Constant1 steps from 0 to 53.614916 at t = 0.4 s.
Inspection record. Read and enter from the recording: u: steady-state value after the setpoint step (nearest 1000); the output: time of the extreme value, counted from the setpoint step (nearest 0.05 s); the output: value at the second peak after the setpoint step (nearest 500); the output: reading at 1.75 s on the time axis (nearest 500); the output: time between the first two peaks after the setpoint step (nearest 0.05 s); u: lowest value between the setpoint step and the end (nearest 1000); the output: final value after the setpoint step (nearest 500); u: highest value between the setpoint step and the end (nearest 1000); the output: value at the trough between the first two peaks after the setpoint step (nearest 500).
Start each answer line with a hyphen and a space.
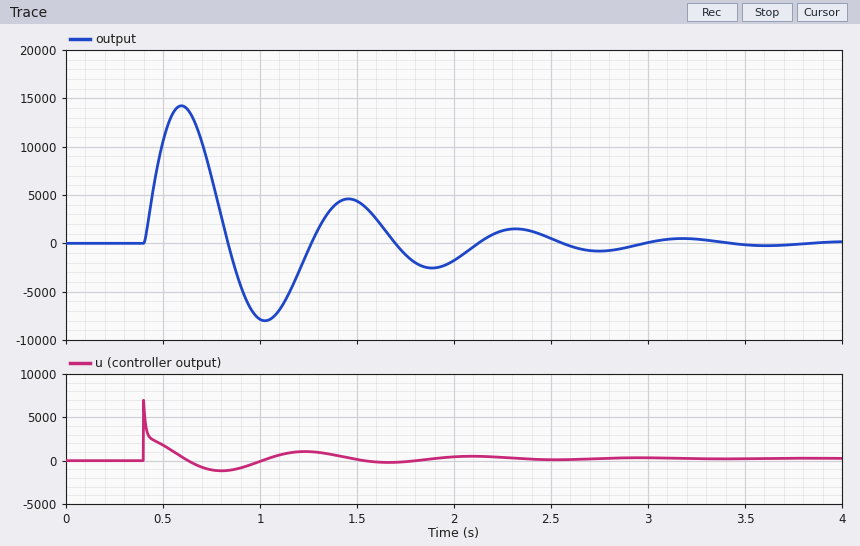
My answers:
- 0
- 0.20 s
- 4500
- -1000
- 0.85 s
- -1000
- 0
- 7000
- -8000
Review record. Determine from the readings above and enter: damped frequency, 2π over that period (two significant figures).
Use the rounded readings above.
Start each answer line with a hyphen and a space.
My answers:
- 7.4 rad/s
